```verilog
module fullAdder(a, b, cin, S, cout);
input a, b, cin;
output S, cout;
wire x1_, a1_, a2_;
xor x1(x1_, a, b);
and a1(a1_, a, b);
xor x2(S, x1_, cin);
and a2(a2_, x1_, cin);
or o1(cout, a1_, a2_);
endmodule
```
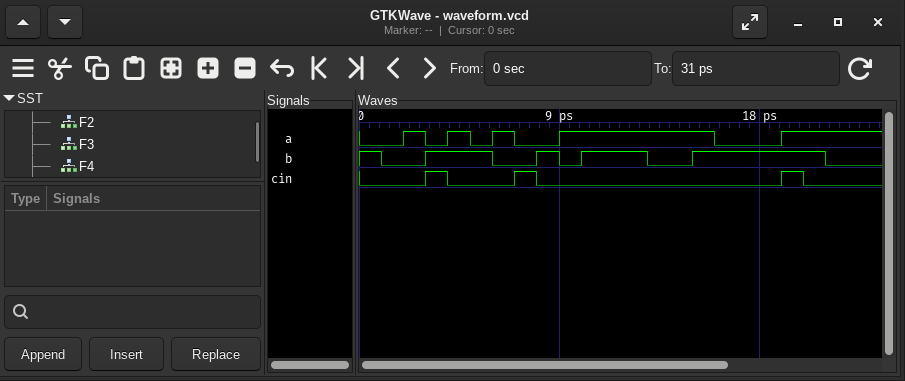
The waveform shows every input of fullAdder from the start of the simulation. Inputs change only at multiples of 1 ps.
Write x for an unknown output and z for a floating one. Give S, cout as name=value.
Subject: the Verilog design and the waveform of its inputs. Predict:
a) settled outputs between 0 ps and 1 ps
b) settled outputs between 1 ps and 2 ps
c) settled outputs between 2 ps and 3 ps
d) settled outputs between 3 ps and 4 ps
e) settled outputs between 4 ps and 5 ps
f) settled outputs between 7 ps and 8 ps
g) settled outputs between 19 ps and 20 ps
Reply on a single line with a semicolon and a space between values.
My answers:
S=1, cout=0; S=0, cout=0; S=1, cout=0; S=0, cout=1; S=0, cout=1; S=1, cout=0; S=1, cout=1
